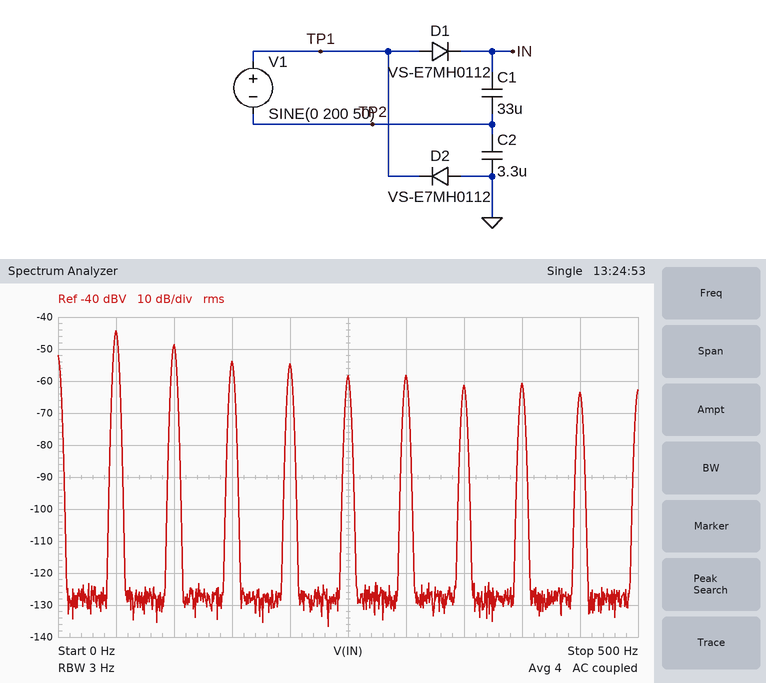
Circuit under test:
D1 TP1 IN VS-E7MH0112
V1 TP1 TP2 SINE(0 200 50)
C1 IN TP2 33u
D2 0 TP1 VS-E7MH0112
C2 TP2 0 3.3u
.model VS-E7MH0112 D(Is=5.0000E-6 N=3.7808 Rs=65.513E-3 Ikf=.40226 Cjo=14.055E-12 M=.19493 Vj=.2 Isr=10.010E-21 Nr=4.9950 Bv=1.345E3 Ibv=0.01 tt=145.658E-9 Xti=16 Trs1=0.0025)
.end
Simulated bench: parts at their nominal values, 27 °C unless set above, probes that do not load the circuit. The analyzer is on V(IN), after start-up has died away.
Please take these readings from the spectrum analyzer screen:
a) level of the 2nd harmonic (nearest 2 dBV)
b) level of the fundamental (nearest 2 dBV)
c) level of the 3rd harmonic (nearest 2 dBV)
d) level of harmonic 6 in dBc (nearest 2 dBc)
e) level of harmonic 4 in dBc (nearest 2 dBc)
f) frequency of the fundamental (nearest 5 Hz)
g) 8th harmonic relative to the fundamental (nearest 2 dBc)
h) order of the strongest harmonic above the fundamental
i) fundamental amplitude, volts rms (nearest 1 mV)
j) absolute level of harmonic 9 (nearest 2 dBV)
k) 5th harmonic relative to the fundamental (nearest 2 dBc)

-48 dBV
-44 dBV
-54 dBV
-14 dBc
-10 dBc
50 Hz
-16 dBc
2
6 mV
-64 dBV
-14 dBc
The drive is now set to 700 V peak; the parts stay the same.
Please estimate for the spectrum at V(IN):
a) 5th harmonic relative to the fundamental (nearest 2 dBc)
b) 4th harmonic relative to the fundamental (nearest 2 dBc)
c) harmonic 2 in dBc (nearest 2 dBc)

-12 dBc
-26 dBc
-24 dBc
